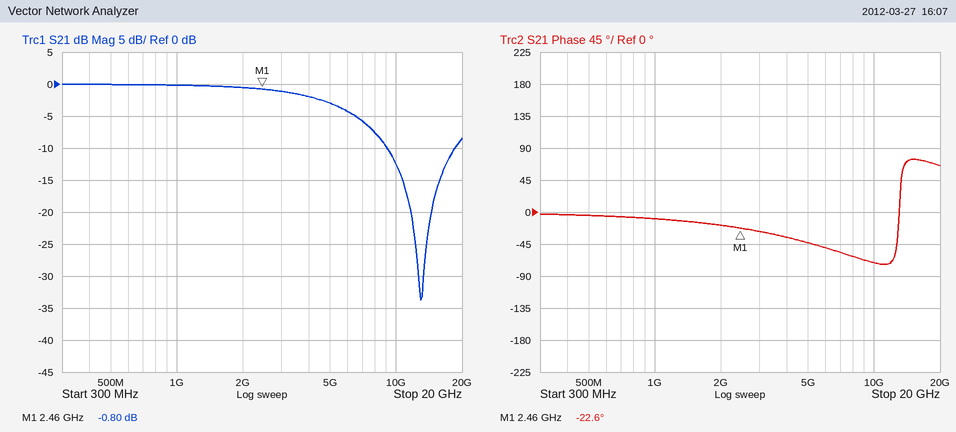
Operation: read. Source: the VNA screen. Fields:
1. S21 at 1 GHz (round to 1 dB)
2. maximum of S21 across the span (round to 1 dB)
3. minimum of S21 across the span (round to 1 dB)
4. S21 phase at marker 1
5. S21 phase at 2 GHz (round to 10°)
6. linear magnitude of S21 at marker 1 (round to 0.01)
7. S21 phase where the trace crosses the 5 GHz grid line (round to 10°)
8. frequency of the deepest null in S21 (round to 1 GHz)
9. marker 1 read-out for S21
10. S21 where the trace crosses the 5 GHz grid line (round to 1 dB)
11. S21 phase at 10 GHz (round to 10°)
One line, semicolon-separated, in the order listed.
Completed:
0 dB; 0 dB; -34 dB; -22.6°; -20°; 0.91; -40°; 13 GHz; -0.80 dB; -3 dB; -70°
